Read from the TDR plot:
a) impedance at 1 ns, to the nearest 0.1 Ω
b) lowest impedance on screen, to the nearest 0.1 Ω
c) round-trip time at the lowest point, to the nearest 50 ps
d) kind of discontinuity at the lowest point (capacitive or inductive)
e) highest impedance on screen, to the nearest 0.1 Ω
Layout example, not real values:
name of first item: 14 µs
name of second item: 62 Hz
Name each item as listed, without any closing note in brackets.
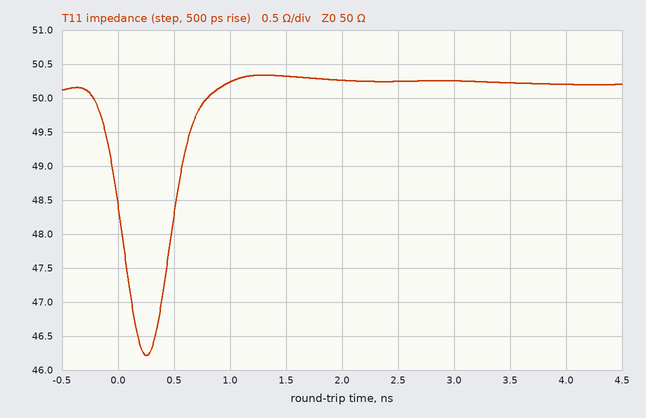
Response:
impedance at 1 ns, to the nearest 0.1 Ω: 50.2 Ω
lowest impedance on screen, to the nearest 0.1 Ω: 46.2 Ω
round-trip time at the lowest point, to the nearest 50 ps: 250 ps
kind of discontinuity at the lowest point: capacitive
highest impedance on screen, to the nearest 0.1 Ω: 50.3 Ω
